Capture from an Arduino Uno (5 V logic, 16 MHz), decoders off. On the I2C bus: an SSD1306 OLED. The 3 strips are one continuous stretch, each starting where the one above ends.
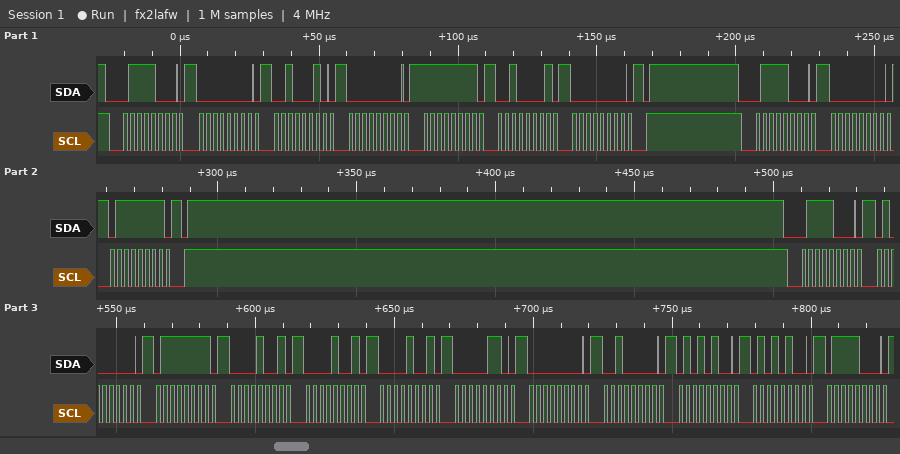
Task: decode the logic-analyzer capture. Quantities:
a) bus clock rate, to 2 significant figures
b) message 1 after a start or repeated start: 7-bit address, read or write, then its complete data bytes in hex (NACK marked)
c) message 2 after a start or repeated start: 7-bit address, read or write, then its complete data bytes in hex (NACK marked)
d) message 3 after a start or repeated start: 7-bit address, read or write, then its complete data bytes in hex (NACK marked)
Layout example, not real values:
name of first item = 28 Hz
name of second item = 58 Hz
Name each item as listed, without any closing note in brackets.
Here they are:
bus clock rate, to 2 significant figures = 400 kHz
message 1 after a start or repeated start: 7-bit address, read or write, then its complete data bytes in hex = 0x3C write: 00 22 00 FF 21 00
message 2 after a start or repeated start: 7-bit address, read or write, then its complete data bytes in hex = 0x3C write: 00 7F
message 3 after a start or repeated start: 7-bit address, read or write, then its complete data bytes in hex = 0x3C write: 40 7F 09 09 09 06 00 20 54 54 78
